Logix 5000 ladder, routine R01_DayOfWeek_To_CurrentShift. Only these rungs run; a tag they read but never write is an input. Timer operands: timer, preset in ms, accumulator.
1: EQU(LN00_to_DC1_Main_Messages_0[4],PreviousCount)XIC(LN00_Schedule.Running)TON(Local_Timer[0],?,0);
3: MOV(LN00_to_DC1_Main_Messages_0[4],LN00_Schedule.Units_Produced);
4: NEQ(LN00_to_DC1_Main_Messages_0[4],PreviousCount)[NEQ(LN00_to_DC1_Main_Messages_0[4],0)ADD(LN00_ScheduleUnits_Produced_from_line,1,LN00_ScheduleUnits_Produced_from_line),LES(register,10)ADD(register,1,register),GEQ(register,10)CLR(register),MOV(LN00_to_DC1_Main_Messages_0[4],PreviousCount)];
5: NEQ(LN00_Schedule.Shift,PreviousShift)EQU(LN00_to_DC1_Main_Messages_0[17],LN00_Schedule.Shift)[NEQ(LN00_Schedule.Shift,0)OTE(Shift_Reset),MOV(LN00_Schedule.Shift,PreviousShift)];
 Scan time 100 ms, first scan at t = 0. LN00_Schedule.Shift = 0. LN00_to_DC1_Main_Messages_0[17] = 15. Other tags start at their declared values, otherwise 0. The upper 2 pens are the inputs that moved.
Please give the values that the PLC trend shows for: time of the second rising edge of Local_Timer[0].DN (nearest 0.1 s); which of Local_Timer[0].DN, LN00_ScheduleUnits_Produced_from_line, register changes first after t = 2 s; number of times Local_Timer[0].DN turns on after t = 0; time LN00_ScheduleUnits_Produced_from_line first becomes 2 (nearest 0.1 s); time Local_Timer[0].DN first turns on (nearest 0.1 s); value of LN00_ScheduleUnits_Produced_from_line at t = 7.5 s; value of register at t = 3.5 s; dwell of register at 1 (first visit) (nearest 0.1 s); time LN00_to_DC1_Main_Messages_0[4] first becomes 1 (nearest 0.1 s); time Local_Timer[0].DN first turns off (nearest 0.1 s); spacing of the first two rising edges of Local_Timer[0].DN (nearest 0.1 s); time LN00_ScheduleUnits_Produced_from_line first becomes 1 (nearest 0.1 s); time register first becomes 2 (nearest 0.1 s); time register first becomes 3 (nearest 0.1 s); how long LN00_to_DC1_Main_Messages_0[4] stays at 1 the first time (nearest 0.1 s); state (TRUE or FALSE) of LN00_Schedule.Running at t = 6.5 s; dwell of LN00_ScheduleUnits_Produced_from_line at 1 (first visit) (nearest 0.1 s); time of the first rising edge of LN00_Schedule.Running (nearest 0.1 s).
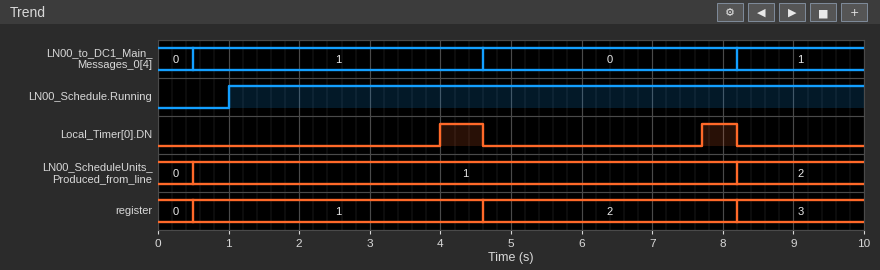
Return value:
7.7 s
Local_Timer[0].DN
2
8.2 s
4.0 s
1
1
4.1 s
0.5 s
4.6 s
3.7 s
0.5 s
4.6 s
8.2 s
4.1 s
TRUE
7.7 s
1.0 s
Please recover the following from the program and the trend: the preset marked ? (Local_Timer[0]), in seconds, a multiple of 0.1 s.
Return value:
3.0 s
